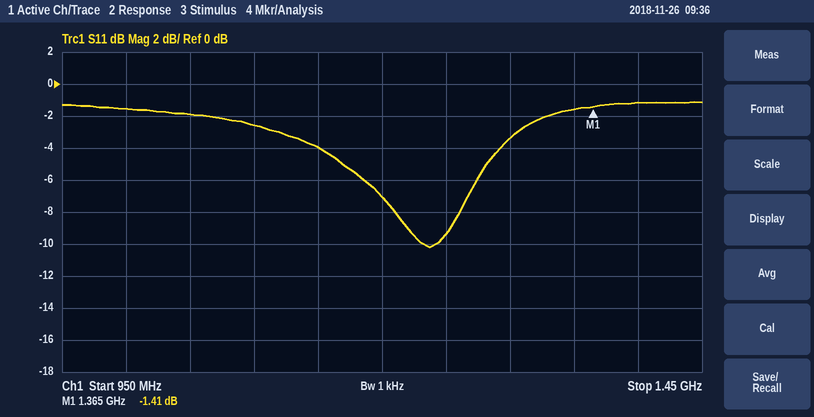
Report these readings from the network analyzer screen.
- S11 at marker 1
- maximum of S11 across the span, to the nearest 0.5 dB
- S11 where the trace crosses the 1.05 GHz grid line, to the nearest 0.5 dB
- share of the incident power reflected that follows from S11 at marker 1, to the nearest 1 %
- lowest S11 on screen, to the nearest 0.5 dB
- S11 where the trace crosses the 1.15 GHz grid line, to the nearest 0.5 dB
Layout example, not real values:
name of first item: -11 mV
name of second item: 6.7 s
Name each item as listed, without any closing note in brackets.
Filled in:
S11 at marker 1: -1.41 dB
maximum of S11 across the span, to the nearest 0.5 dB: -1.0 dB
S11 where the trace crosses the 1.05 GHz grid line, to the nearest 0.5 dB: -2.0 dB
share of the incident power reflected that follows from S11 at marker 1, to the nearest 1 %: 72 %
lowest S11 on screen, to the nearest 0.5 dB: -10.0 dB
S11 where the trace crosses the 1.15 GHz grid line, to the nearest 0.5 dB: -4.0 dB
